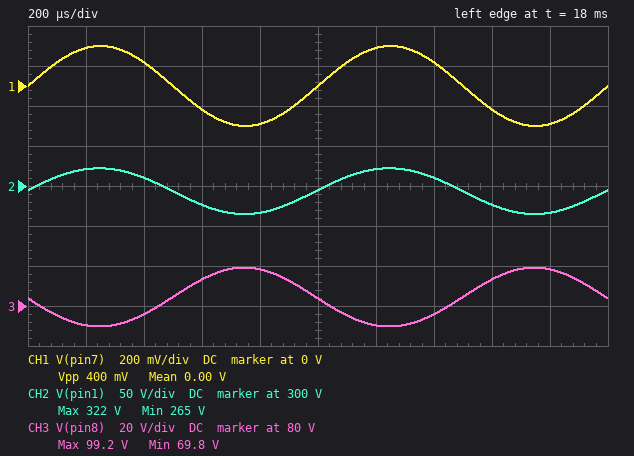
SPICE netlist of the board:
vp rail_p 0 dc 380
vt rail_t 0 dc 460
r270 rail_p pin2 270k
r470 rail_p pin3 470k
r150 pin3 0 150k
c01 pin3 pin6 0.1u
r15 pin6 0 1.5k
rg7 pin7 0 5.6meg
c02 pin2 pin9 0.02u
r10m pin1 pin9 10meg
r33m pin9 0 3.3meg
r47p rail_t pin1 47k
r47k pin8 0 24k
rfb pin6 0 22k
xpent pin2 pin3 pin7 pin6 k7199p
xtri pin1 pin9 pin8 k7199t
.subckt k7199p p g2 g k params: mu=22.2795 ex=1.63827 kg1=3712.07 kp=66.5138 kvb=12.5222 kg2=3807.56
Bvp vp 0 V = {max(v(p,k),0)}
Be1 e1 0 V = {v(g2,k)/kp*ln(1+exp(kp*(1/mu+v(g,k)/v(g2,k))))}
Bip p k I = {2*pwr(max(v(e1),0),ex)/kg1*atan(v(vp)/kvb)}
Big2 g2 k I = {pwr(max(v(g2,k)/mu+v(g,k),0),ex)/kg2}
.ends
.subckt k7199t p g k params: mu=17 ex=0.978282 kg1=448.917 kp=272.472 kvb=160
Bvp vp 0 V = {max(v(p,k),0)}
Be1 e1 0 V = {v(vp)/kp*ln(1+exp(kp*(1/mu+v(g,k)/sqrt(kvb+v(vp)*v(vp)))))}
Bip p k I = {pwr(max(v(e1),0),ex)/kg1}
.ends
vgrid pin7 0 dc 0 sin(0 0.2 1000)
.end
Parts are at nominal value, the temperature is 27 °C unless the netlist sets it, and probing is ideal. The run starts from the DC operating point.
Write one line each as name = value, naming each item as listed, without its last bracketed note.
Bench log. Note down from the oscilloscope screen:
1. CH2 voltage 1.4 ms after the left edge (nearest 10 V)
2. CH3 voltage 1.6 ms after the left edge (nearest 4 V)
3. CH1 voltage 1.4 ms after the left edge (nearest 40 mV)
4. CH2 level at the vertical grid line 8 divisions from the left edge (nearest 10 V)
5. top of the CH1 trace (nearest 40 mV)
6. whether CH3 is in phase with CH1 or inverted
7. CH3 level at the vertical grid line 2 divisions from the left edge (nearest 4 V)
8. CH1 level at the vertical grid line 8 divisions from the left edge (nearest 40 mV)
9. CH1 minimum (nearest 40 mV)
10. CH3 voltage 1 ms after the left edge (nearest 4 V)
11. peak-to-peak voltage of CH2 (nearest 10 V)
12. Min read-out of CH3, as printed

CH2 voltage 1.4 ms after the left edge = 310 V
CH3 voltage 1.6 ms after the left edge = 92 V
CH1 voltage 1.4 ms after the left edge = 120 mV
CH2 level at the vertical grid line 8 divisions from the left edge = 280 V
top of the CH1 trace = 200 mV
whether CH3 is in phase with CH1 or inverted = inverted
CH3 level at the vertical grid line 2 divisions from the left edge = 76 V
CH1 level at the vertical grid line 8 divisions from the left edge = -120 mV
CH1 minimum = -200 mV
CH3 voltage 1 ms after the left edge = 84 V
peak-to-peak voltage of CH2 = 60 V
Min read-out of CH3, as printed = 69.8 V
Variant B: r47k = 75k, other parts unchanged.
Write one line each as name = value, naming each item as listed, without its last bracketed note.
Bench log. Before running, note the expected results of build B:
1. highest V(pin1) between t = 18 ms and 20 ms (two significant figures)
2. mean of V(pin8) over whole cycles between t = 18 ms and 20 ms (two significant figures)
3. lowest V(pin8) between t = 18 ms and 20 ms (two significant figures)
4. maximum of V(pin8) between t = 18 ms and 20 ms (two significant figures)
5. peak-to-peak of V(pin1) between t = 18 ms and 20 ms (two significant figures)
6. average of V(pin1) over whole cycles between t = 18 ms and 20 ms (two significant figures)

highest V(pin1) between t = 18 ms and 20 ms = 400 V
mean of V(pin8) over whole cycles between t = 18 ms and 20 ms = 110 V
lowest V(pin8) between t = 18 ms and 20 ms = 97 V
maximum of V(pin8) between t = 18 ms and 20 ms = 130 V
peak-to-peak of V(pin1) between t = 18 ms and 20 ms = 20 V
average of V(pin1) over whole cycles between t = 18 ms and 20 ms = 390 V
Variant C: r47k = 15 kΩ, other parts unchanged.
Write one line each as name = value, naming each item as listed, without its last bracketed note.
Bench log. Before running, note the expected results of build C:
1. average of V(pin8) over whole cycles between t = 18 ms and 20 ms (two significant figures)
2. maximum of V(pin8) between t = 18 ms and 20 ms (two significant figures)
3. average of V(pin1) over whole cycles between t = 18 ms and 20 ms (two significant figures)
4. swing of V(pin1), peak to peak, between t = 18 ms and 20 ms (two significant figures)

average of V(pin8) over whole cycles between t = 18 ms and 20 ms = 69 V
maximum of V(pin8) between t = 18 ms and 20 ms = 83 V
average of V(pin1) over whole cycles between t = 18 ms and 20 ms = 240 V
swing of V(pin1), peak to peak, between t = 18 ms and 20 ms = 85 V
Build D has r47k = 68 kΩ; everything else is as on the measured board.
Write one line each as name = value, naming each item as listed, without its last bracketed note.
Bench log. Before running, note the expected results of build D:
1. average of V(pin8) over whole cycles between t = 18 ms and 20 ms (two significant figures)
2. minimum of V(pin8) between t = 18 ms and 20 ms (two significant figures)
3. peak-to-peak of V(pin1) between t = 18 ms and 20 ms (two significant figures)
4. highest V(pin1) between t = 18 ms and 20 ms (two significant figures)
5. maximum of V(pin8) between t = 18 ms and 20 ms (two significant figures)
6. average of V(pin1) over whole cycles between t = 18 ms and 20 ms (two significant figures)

average of V(pin8) over whole cycles between t = 18 ms and 20 ms = 110 V
minimum of V(pin8) between t = 18 ms and 20 ms = 95 V
peak-to-peak of V(pin1) between t = 18 ms and 20 ms = 22 V
highest V(pin1) between t = 18 ms and 20 ms = 390 V
maximum of V(pin8) between t = 18 ms and 20 ms = 130 V
average of V(pin1) over whole cycles between t = 18 ms and 20 ms = 380 V
